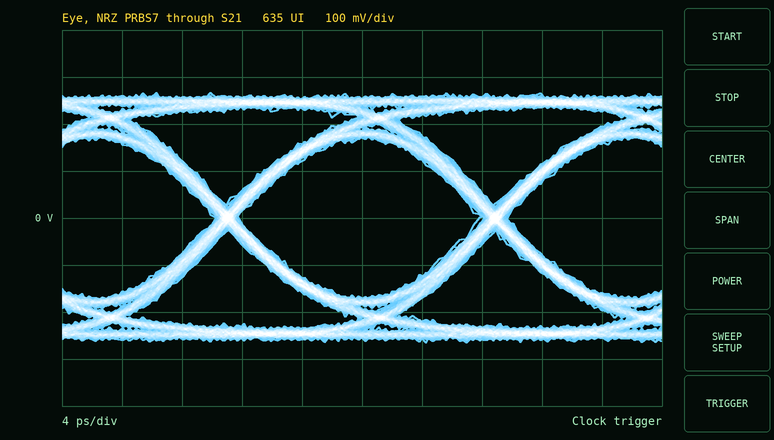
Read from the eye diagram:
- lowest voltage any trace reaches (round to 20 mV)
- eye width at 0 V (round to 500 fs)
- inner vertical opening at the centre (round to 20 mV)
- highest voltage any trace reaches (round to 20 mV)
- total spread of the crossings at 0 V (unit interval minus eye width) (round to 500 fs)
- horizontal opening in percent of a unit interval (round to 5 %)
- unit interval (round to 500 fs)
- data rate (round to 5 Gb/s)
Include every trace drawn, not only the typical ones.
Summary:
-260 mV
16.0 ps
340 mV
260 mV
2.0 ps
90 %
18.0 ps
55 Gb/s
